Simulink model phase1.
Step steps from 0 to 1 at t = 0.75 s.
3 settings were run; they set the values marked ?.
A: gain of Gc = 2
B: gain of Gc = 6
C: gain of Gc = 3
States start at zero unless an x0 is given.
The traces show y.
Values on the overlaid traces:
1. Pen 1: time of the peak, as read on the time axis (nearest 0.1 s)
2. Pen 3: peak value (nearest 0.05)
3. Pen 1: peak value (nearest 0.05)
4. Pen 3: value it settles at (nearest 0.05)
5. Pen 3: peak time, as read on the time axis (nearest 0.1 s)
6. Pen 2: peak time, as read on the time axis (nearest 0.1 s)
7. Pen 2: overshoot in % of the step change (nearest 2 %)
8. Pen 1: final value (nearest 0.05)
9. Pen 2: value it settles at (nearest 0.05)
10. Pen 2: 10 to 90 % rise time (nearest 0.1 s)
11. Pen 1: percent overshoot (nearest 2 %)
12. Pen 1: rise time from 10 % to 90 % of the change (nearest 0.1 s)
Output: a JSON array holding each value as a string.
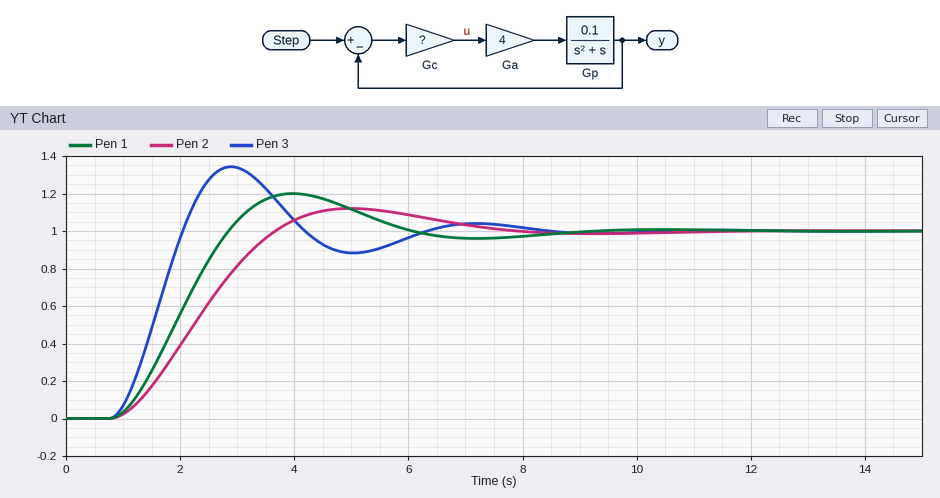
["4.0 s", "1.35", "1.20", "1.00", "2.9 s", "5.0 s", "12 %", "1.00", "1.00", "2.0 s", "20 %", "1.4 s"]
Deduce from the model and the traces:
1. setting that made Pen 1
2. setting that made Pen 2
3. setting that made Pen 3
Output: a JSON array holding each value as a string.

["C", "A", "B"]
